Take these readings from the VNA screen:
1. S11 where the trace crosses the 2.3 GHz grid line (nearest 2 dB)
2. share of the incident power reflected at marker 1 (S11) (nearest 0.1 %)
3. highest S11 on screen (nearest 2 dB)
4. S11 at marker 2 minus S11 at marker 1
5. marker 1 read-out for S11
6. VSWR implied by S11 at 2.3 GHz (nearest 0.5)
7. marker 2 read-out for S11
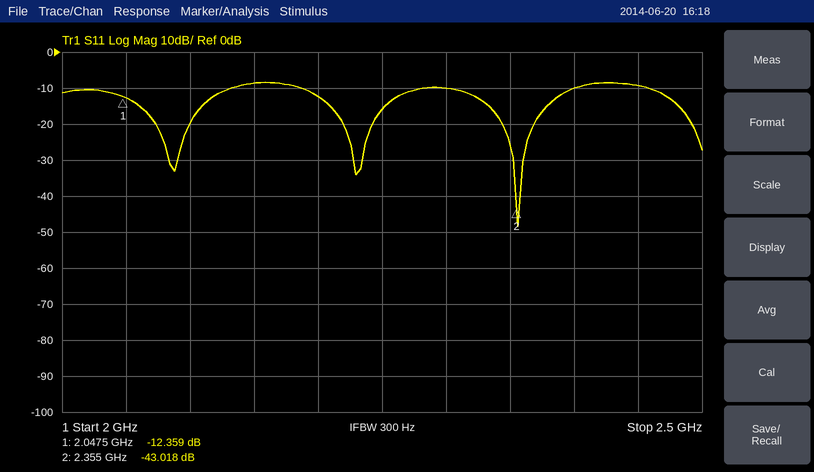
-10 dB
5.8 %
-8 dB
-30.659 dB
-12.359 dB
2.0
-43.018 dB
